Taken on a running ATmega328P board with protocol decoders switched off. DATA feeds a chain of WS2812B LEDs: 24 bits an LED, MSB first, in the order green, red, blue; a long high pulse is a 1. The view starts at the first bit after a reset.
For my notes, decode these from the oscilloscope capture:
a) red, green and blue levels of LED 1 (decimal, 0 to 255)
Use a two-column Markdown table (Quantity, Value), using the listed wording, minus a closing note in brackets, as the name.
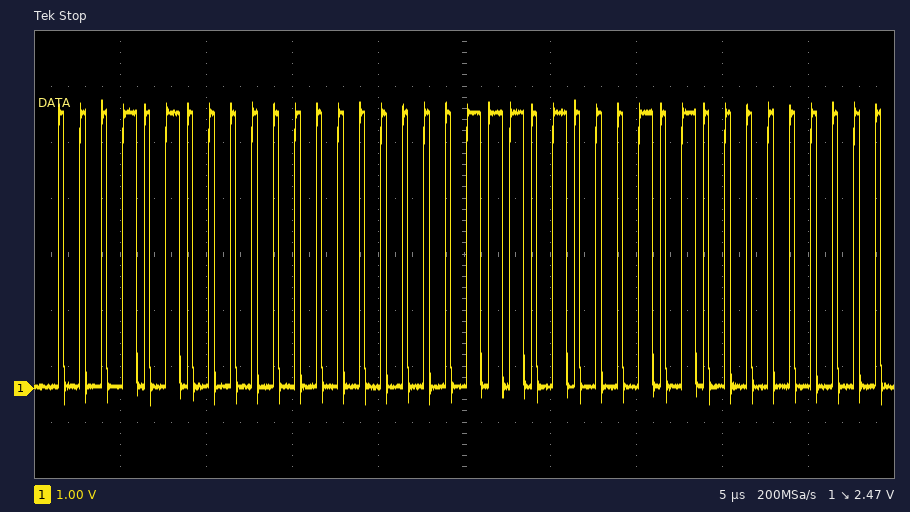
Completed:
| Quantity | Value |
|---|---|
| red, green and blue levels of LED 1 | 0, 20, 29 |
